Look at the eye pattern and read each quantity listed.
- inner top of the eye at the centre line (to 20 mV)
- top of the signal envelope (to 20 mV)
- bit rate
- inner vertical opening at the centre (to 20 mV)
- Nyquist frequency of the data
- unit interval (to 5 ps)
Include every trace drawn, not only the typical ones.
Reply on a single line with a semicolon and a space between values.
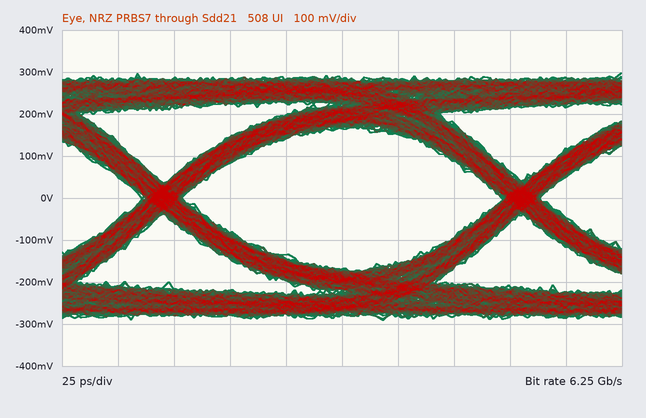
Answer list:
160 mV; 300 mV; 6.25 Gb/s; 340 mV; 3.125 GHz; 160 ps
